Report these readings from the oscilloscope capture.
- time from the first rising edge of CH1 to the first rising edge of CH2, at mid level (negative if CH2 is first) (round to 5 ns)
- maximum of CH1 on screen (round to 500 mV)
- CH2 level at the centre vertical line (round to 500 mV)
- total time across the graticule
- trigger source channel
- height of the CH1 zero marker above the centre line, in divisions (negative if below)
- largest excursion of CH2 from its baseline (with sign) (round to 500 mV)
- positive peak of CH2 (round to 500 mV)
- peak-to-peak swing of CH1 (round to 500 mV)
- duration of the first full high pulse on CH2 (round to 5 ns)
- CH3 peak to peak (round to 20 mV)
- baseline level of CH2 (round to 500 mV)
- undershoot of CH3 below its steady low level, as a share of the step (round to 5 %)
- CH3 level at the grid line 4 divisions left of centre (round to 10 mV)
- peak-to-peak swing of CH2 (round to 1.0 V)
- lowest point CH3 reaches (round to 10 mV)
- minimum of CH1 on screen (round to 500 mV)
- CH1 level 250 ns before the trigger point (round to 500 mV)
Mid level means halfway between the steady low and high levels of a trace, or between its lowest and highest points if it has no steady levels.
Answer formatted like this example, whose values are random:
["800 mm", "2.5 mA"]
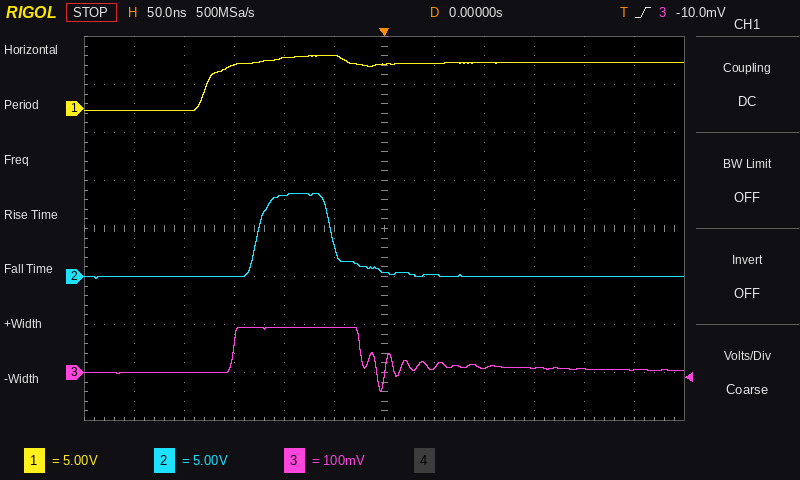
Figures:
["+50 ns", "5.5 V", "500 mV", "600 ns", "CH3", "+2.5 div", "+8.5 V", "8.5 V", "5.5 V", "75 ns", "140 mV", "0.0 V", "50 %", "0 mV", "9.0 V", "-40 mV", "0.0 V", "0.0 V"]
